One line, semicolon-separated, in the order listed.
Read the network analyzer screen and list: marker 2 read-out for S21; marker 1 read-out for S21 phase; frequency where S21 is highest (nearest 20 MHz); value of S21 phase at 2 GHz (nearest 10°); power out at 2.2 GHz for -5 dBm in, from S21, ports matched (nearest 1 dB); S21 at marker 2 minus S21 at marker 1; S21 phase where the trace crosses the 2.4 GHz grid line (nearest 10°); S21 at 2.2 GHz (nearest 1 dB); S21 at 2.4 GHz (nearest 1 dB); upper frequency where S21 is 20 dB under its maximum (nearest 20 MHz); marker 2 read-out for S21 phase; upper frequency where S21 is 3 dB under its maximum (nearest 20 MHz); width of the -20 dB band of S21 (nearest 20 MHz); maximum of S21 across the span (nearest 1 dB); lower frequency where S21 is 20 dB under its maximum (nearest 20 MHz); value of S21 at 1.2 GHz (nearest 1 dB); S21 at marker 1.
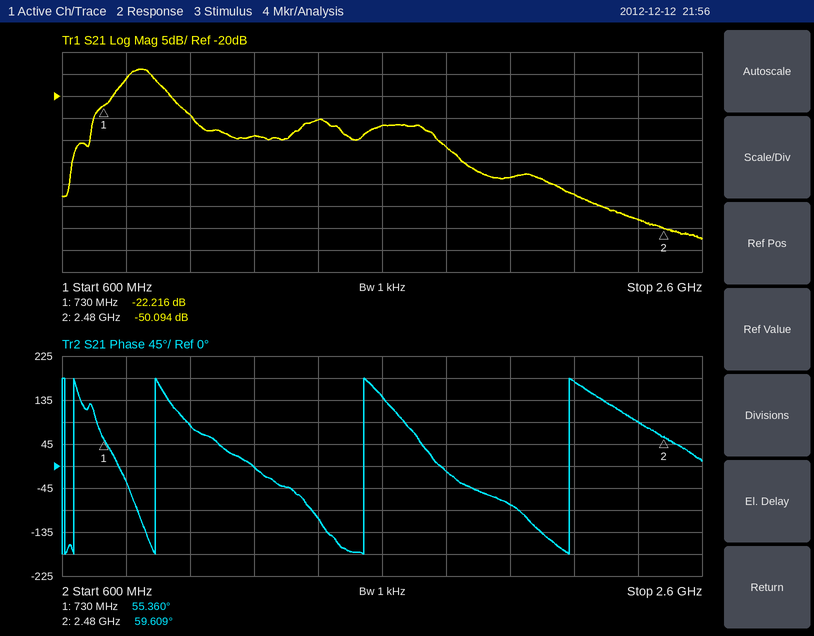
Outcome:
-50.094 dB; 55.360°; 840 MHz; -80°; -47 dBm; -27.878 dB; 90°; -42 dB; -48 dB; 1.84 GHz; 59.609°; 900 MHz; 1.20 GHz; -14 dB; 640 MHz; -29 dB; -22.216 dB
